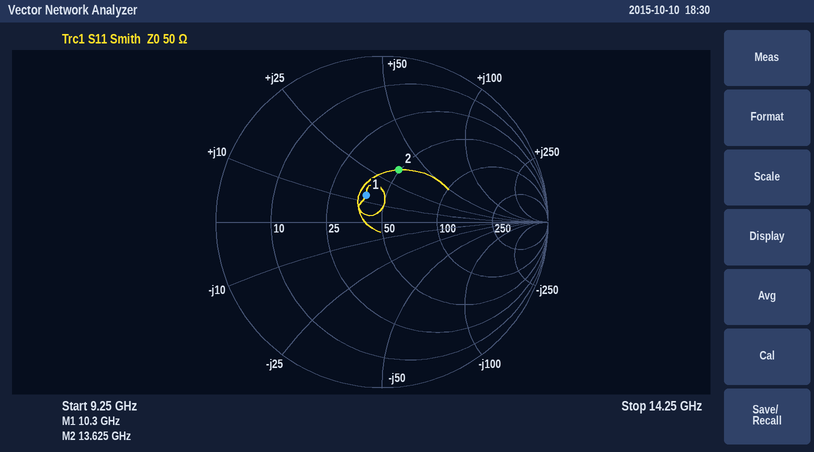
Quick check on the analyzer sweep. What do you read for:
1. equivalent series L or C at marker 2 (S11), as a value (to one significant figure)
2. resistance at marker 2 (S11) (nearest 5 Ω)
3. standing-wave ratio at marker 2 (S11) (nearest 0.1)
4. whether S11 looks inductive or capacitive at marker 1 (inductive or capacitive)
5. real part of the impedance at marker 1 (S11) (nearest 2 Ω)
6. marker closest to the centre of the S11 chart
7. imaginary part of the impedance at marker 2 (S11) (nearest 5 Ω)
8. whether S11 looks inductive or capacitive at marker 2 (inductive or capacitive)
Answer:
400 pH
50 Ω
2.0
inductive
40 Ω
marker 1
+35 Ω
inductive
